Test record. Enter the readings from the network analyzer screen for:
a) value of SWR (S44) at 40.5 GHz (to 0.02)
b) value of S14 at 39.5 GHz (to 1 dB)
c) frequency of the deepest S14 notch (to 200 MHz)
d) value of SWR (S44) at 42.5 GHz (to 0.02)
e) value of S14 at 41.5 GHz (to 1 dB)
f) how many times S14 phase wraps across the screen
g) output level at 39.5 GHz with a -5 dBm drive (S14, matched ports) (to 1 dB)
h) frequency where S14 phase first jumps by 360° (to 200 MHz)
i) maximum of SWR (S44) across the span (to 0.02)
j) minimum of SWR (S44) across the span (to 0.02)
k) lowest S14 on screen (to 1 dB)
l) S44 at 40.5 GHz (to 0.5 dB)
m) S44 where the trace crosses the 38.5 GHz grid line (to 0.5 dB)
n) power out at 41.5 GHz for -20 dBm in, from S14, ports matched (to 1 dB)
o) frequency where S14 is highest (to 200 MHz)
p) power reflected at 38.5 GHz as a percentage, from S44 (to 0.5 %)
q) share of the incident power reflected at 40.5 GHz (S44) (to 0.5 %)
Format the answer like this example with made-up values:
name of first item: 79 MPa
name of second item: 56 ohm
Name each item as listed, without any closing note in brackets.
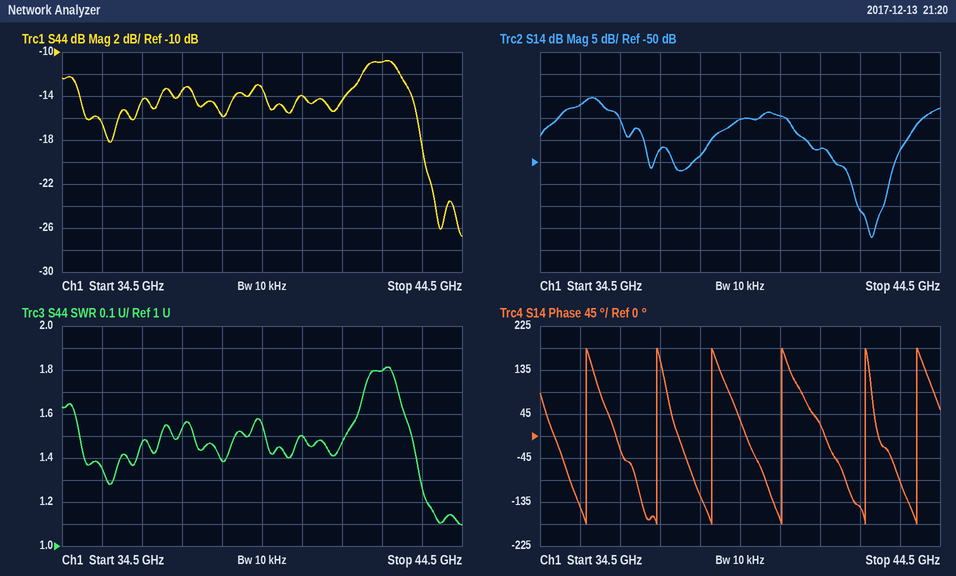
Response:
value of SWR (S44) at 40.5 GHz: 1.50
value of S14 at 39.5 GHz: -40 dB
frequency of the deepest S14 notch: 42.8 GHz
value of SWR (S44) at 42.5 GHz: 1.80
value of S14 at 41.5 GHz: -47 dB
how many times S14 phase wraps across the screen: 6
output level at 39.5 GHz with a -5 dBm drive (S14, matched ports): -45 dBm
frequency where S14 phase first jumps by 360°: 35.6 GHz
maximum of SWR (S44) across the span: 1.82
minimum of SWR (S44) across the span: 1.10
lowest S14 on screen: -67 dB
S44 at 40.5 GHz: -14.0 dB
S44 where the trace crosses the 38.5 GHz grid line: -16.0 dB
power out at 41.5 GHz for -20 dBm in, from S14, ports matched: -67 dBm
frequency where S14 is highest: 35.8 GHz
power reflected at 38.5 GHz as a percentage, from S44: 2.5 %
share of the incident power reflected at 40.5 GHz (S44): 4.0 %
